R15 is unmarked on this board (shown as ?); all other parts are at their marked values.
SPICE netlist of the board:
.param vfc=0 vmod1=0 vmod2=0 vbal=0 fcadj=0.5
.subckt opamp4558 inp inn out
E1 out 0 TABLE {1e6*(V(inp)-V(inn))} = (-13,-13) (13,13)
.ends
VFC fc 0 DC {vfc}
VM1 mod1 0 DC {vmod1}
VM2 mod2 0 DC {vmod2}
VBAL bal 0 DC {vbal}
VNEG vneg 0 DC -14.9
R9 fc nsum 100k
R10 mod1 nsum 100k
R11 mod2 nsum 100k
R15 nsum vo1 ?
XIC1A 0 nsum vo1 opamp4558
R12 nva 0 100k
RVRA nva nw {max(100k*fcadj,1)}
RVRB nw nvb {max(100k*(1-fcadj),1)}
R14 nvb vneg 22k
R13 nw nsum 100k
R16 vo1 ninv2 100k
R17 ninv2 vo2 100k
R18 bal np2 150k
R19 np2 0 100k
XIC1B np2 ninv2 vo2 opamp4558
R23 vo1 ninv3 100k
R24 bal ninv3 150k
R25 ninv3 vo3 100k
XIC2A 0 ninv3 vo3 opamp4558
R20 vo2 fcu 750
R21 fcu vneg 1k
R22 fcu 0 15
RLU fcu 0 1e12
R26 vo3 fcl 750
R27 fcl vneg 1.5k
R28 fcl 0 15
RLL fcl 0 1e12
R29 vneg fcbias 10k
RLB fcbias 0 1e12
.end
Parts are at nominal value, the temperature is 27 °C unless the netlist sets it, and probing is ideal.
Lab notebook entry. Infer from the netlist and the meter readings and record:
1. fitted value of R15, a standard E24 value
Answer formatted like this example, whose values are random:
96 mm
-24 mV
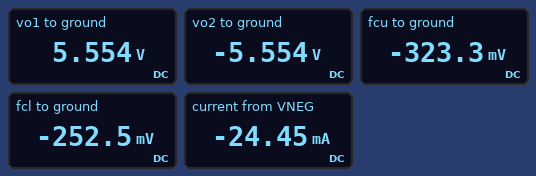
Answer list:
82 kΩ
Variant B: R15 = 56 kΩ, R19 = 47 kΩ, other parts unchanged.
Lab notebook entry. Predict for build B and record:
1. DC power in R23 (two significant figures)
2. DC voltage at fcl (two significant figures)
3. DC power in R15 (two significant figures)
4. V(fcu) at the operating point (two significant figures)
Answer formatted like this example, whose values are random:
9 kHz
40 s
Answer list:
140 µW
-220 mV
260 µW
-290 mV
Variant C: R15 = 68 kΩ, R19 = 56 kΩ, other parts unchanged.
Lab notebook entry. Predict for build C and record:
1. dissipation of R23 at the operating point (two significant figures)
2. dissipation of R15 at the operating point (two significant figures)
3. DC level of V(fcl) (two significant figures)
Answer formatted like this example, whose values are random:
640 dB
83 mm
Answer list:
210 µW
310 µW
-230 mV
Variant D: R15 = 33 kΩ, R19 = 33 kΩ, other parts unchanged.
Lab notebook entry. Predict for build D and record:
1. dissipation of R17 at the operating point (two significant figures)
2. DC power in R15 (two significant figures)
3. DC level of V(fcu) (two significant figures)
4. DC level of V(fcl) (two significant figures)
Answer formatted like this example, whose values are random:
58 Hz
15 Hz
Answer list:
50 µW
150 µW
-260 mV
-190 mV
